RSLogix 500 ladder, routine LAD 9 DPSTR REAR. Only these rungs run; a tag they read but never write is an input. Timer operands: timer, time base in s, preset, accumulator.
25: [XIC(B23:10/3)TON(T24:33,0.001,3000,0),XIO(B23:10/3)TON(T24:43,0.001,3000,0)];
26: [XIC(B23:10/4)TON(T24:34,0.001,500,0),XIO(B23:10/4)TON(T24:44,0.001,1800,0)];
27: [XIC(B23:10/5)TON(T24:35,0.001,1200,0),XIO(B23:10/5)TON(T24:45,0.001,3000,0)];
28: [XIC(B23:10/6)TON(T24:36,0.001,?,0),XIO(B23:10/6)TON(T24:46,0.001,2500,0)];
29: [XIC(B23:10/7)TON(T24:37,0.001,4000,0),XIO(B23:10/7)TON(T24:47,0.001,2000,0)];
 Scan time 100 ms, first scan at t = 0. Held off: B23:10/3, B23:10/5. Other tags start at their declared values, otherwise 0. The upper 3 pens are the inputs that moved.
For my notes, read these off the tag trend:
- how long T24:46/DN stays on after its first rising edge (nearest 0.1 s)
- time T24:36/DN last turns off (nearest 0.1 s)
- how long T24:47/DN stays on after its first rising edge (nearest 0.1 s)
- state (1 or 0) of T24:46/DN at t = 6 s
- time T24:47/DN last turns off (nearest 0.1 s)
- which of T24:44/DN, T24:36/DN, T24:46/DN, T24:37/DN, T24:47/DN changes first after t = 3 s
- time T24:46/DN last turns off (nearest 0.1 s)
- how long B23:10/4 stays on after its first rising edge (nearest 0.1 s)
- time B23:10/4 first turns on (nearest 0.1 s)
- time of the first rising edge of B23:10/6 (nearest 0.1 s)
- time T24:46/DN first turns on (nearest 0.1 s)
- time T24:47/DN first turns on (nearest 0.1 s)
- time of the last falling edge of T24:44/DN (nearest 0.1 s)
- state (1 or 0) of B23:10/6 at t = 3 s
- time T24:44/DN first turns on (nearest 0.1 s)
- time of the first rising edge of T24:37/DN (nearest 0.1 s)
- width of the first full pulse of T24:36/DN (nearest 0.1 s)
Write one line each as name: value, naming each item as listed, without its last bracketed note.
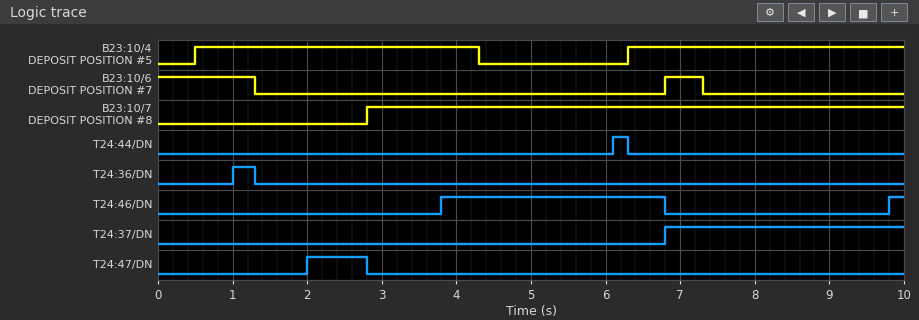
how long T24:46/DN stays on after its first rising edge: 3.0 s
time T24:36/DN last turns off: 1.3 s
how long T24:47/DN stays on after its first rising edge: 0.8 s
state (1 or 0) of T24:46/DN at t = 6 s: 1
time T24:47/DN last turns off: 2.8 s
which of T24:44/DN, T24:36/DN, T24:46/DN, T24:37/DN, T24:47/DN changes first after t = 3 s: T24:46/DN
time T24:46/DN last turns off: 6.8 s
how long B23:10/4 stays on after its first rising edge: 3.8 s
time B23:10/4 first turns on: 0.5 s
time of the first rising edge of B23:10/6: 6.8 s
time T24:46/DN first turns on: 3.8 s
time T24:47/DN first turns on: 2.0 s
time of the last falling edge of T24:44/DN: 6.3 s
state (1 or 0) of B23:10/6 at t = 3 s: 0
time T24:44/DN first turns on: 6.1 s
time of the first rising edge of T24:37/DN: 6.8 s
width of the first full pulse of T24:36/DN: 0.3 s
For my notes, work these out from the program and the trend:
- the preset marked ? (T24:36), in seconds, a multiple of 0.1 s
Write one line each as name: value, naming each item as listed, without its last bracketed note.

the preset marked ? (T24:36), in seconds, a multiple of 0.1 s: 1.0 s
